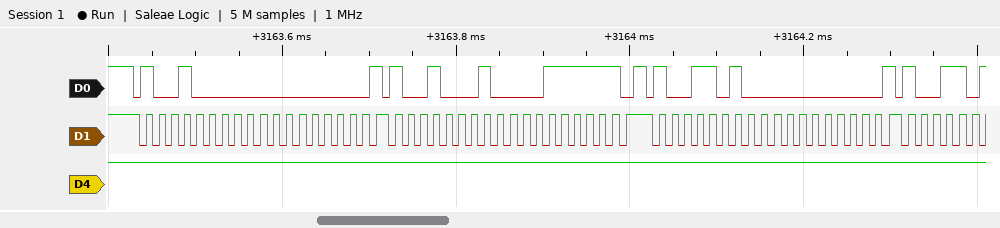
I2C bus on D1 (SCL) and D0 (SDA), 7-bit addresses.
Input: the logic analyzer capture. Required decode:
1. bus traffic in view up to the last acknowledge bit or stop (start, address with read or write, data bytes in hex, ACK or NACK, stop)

start, address 48 write ACK, 00 ACK, repeated start, address 48 read ACK, 1F NACK, stop, start, address 4D write ACK, 00 ACK
